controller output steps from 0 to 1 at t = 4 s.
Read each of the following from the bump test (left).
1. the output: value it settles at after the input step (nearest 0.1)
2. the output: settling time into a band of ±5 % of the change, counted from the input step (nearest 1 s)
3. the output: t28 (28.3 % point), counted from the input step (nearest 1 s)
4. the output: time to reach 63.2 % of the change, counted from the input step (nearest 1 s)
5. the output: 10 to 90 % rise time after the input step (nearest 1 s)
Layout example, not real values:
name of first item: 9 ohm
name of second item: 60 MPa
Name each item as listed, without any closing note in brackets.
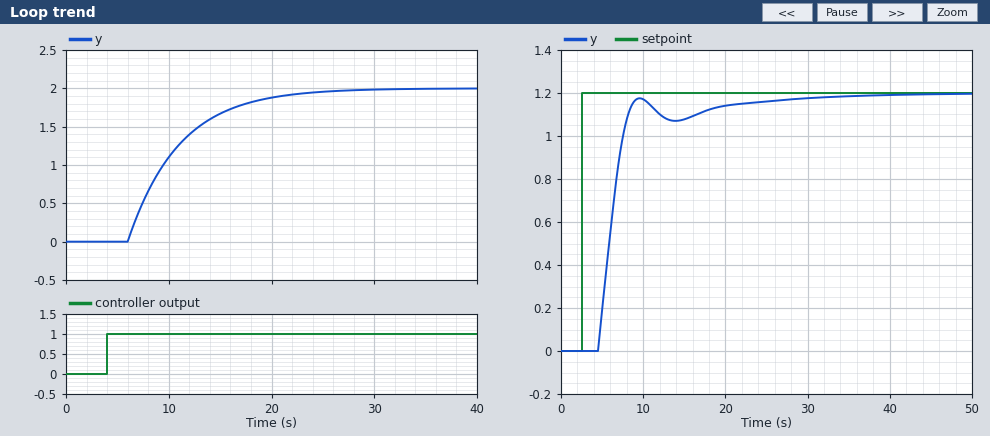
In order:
the output: value it settles at after the input step: 2.0
the output: settling time into a band of ±5 % of the change, counted from the input step: 17 s
the output: t28 (28.3 % point), counted from the input step: 4 s
the output: time to reach 63.2 % of the change, counted from the input step: 7 s
the output: 10 to 90 % rise time after the input step: 11 s
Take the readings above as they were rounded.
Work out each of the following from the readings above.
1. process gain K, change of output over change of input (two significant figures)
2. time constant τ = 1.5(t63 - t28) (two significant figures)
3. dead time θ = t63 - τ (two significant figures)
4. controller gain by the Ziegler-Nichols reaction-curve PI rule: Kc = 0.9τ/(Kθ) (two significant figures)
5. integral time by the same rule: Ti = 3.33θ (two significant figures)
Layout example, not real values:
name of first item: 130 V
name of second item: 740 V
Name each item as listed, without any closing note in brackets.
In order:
process gain K, change of output over change of input: 2.0
time constant τ = 1.5(t63 - t28): 4.5 s
dead time θ = t63 - τ: 2.5 s
controller gain by the Ziegler-Nichols reaction-curve PI rule: Kc = 0.9τ/(Kθ): 0.81
integral time by the same rule: Ti = 3.33θ: 8.3 s
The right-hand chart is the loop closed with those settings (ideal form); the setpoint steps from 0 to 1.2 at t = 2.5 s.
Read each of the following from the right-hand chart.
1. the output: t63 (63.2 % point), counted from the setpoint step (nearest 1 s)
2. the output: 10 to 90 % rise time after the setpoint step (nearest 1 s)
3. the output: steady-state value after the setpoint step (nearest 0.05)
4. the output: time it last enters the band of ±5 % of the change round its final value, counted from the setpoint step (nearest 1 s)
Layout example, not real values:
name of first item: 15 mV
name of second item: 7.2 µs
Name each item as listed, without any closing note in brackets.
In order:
the output: t63 (63.2 % point), counted from the setpoint step: 4 s
the output: 10 to 90 % rise time after the setpoint step: 3 s
the output: steady-state value after the setpoint step: 1.20
the output: time it last enters the band of ±5 % of the change round its final value, counted from the setpoint step: 17 s
